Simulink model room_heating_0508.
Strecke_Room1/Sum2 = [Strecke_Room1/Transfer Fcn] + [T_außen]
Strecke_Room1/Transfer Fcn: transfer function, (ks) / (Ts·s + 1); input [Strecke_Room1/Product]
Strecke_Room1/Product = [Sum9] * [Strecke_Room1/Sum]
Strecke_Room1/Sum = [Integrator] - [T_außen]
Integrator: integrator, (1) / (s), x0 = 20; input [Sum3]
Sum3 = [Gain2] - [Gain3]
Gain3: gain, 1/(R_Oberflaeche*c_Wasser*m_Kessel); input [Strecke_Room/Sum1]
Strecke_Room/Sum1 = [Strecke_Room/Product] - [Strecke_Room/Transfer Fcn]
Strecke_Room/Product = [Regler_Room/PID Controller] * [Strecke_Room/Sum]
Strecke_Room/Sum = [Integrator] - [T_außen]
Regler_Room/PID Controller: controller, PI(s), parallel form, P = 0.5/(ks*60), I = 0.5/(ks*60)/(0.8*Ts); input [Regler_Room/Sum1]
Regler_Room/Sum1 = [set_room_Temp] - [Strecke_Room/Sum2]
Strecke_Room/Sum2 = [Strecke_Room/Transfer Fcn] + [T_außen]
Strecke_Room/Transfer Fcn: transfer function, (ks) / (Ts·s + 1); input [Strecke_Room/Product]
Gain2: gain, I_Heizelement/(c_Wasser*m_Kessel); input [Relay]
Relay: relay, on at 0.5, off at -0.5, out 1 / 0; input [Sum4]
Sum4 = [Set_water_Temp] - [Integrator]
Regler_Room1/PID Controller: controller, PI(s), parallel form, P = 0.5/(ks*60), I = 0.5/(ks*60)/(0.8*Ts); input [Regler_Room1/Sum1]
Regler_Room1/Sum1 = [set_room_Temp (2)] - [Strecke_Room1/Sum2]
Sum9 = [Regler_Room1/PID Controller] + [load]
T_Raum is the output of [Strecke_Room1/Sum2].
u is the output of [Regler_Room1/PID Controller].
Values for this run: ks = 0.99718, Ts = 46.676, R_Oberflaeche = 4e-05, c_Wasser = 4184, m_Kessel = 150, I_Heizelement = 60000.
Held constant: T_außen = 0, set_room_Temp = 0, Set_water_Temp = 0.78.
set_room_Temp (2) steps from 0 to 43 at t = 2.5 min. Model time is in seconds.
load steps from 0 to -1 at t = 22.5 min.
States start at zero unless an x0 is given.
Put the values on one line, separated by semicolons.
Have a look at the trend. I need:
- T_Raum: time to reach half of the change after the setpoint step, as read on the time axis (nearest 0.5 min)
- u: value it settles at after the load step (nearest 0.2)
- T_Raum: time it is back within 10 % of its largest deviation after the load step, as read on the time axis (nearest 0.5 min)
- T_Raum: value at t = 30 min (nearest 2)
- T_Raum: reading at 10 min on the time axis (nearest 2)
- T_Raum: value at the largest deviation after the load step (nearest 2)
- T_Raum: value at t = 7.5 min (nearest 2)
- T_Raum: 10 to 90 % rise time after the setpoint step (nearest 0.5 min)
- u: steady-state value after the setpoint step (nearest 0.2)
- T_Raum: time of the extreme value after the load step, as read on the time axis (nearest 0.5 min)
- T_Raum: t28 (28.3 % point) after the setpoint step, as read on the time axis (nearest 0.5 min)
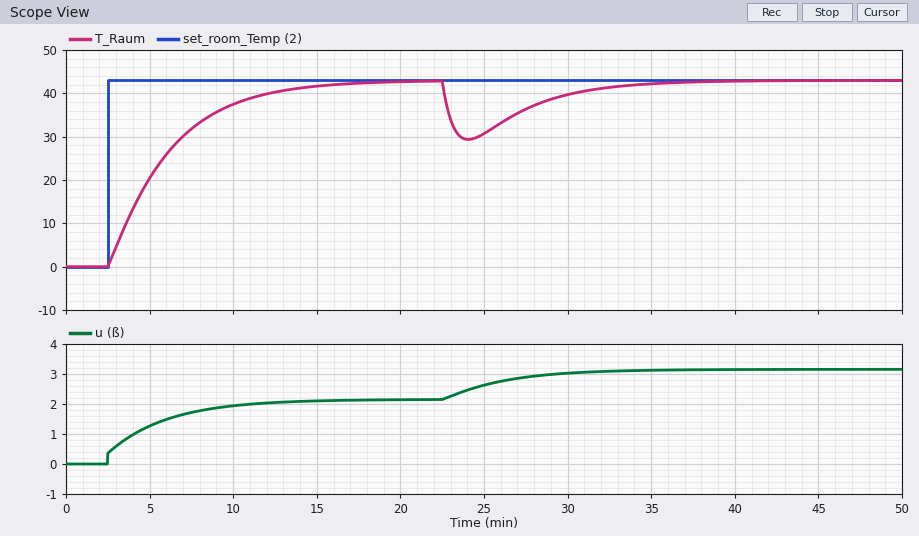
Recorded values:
5.0 min; 3.2; 33.0 min; 40; 38; 30; 32; 8.0 min; 2.2; 24.0 min; 4.0 min
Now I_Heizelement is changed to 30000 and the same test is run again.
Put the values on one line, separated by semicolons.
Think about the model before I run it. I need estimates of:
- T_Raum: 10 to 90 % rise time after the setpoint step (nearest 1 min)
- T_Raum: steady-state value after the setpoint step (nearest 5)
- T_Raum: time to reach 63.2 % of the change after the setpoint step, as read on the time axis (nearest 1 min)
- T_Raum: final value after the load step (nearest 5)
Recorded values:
8 min; 45; 6 min; 45
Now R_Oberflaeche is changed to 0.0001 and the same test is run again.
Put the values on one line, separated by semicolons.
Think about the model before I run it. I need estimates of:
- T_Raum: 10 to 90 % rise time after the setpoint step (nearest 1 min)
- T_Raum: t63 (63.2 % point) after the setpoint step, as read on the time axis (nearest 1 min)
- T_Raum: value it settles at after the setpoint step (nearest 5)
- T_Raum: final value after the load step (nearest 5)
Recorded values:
8 min; 6 min; 45; 45
